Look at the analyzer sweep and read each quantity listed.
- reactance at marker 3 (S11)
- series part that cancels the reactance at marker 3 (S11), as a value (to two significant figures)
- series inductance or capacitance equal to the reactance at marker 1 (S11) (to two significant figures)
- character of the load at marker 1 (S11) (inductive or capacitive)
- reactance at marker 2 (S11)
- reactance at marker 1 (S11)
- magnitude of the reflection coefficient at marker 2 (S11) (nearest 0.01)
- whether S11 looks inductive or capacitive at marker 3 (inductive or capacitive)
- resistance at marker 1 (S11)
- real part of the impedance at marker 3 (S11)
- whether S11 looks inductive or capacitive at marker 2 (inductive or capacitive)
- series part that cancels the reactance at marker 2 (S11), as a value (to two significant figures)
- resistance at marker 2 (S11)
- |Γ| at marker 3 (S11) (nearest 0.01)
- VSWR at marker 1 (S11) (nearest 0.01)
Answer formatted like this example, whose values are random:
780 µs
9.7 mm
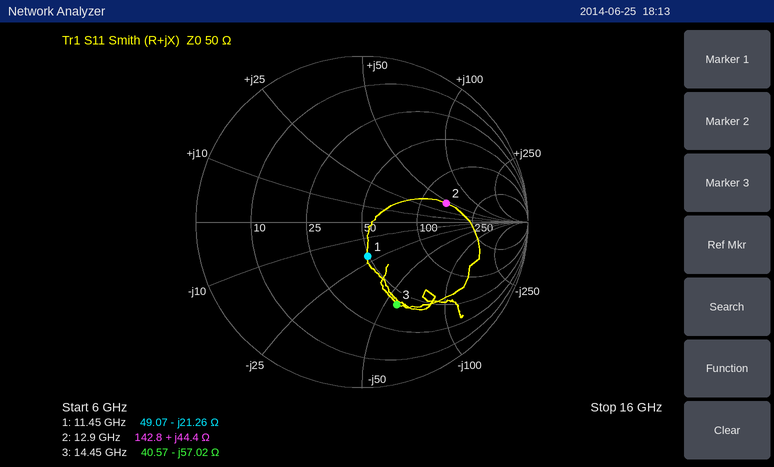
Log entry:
-57.02 Ω
630 pH
650 fF
capacitive
+44.4 Ω
-21.26 Ω
0.52
capacitive
49.07 Ω
40.57 Ω
inductive
280 fF
142.8 Ω
0.54
1.53
